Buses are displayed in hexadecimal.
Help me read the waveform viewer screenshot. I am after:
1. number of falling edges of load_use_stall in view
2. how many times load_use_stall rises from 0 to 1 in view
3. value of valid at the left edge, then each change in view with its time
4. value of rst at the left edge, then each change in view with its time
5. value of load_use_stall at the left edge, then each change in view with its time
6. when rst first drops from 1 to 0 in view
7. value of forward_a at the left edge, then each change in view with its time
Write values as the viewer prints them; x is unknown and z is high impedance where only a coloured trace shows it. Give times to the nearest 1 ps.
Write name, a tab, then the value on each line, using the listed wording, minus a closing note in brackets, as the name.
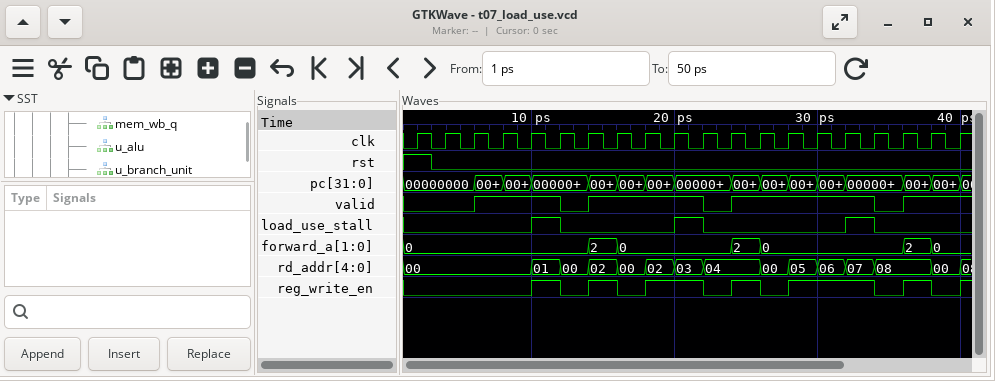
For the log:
number of falling edges of load_use_stall in view	3
how many times load_use_stall rises from 0 to 1 in view	3
value of valid at the left edge, then each change in view with its time	0, 1 at 6 ps, 0 at 12 ps, 1 at 14 ps, 0 at 22 ps, 1 at 24 ps, 0 at 34 ps, 1 at 36 ps
value of rst at the left edge, then each change in view with its time	1, 0 at 3 ps
value of load_use_stall at the left edge, then each change in view with its time	0, 1 at 10 ps, 0 at 12 ps, 1 at 20 ps, 0 at 22 ps, 1 at 32 ps, 0 at 34 ps
when rst first drops from 1 to 0 in view	3 ps
value of forward_a at the left edge, then each change in view with its time	0, 2 at 14 ps, 0 at 16 ps, 2 at 24 ps, 0 at 26 ps, 2 at 36 ps, 0 at 38 ps
